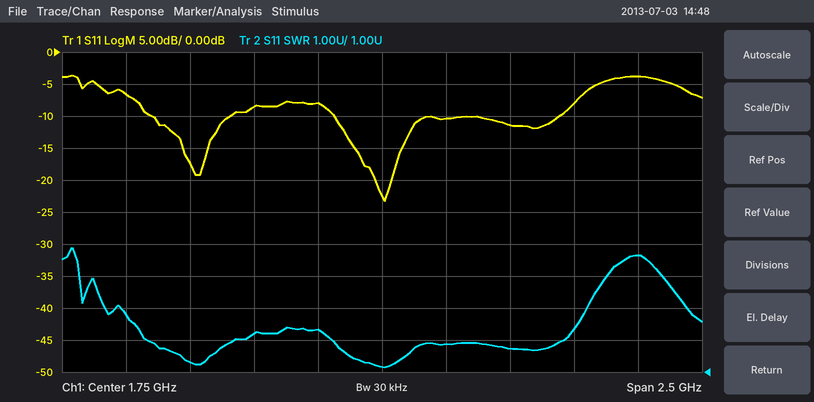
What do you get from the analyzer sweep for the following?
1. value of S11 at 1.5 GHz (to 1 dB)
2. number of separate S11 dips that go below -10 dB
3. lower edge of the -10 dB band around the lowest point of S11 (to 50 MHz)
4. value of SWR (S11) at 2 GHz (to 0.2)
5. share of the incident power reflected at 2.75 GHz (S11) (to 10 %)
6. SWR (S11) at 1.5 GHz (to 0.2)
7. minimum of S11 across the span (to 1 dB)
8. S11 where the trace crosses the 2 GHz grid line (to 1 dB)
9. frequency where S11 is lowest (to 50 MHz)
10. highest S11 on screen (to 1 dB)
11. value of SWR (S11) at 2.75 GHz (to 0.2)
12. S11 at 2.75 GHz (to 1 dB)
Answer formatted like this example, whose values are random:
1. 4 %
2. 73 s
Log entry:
1. -8 dB
2. 2
3. 1.55 GHz
4. 1.8
5. 40 %
6. 2.4
7. -23 dB
8. -10 dB
9. 1.75 GHz
10. -4 dB
11. 4.6
12. -4 dB
